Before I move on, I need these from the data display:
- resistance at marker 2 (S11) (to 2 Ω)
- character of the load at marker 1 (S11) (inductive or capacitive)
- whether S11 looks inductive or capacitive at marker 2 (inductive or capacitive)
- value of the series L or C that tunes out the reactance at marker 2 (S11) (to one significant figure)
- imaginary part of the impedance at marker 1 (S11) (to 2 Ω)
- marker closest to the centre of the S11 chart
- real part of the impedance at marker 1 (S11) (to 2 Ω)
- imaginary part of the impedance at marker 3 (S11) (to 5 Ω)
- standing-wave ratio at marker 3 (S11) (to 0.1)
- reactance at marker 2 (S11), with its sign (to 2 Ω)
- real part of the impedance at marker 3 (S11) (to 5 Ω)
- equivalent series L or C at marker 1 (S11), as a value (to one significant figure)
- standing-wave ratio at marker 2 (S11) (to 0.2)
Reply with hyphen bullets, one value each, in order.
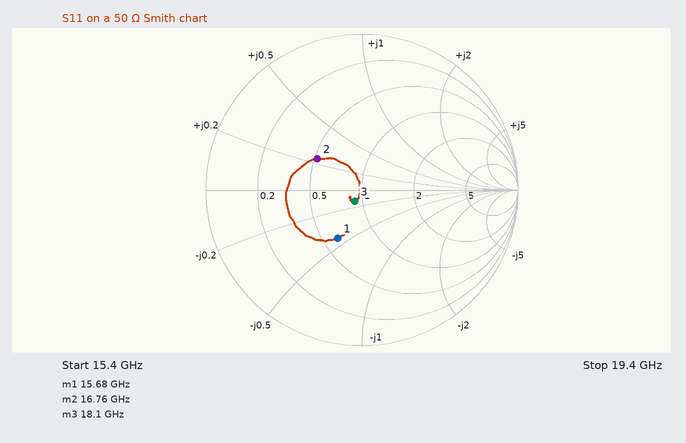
- 26 Ω
- capacitive
- inductive
- 800 fF
- -22 Ω
- marker 3
- 30 Ω
- -5 Ω
- 1.2
- +12 Ω
- 45 Ω
- 500 fF
- 2.0
